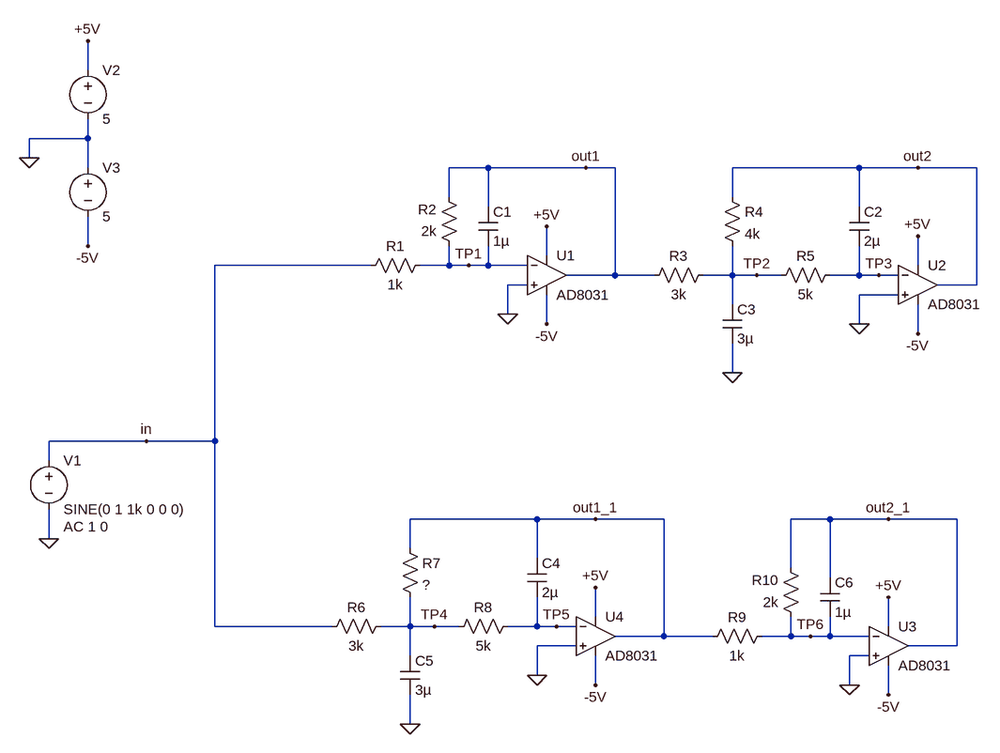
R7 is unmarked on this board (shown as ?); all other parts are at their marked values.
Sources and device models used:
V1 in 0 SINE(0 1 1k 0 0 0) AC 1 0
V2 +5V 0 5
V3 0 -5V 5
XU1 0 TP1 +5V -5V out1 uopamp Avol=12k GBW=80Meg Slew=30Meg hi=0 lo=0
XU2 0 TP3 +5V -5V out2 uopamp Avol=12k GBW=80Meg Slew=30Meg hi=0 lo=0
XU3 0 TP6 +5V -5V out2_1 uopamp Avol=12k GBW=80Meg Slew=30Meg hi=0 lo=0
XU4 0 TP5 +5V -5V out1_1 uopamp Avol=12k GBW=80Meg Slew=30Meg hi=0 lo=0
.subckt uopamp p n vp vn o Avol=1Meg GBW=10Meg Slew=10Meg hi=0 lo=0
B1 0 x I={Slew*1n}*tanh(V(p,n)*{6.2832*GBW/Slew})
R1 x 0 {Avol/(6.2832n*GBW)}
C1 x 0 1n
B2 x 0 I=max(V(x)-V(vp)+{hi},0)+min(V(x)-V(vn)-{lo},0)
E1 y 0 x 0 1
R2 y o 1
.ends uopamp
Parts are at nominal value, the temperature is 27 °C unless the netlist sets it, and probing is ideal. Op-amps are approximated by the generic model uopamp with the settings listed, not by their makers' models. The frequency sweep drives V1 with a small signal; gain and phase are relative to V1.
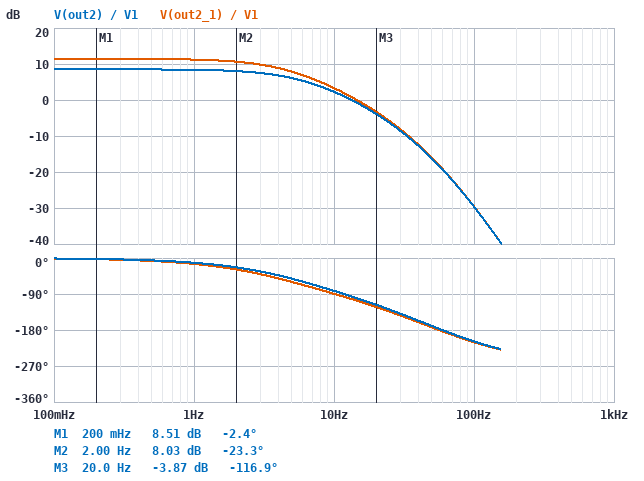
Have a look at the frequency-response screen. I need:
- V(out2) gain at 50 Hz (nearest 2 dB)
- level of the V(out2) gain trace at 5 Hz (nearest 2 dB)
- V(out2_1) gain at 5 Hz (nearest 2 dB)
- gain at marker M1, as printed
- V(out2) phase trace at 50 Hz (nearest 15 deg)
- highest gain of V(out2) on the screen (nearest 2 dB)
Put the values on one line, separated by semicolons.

-16 dB; 6 dB; 8 dB; 8.51 dB; -165 deg; 8 dB
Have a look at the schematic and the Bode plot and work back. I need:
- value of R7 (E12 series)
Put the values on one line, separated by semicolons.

5.6 kΩ
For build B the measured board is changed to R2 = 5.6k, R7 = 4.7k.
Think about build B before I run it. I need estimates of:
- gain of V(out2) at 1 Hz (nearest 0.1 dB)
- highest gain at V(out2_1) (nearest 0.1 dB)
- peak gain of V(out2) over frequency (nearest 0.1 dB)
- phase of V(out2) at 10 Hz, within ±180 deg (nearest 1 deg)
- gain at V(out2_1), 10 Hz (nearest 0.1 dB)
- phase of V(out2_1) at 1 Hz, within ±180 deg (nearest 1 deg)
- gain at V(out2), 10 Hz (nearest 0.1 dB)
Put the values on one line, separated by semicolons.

17.3 dB; 9.9 dB; 17.5 dB; -94 deg; 2.8 dB; -13 deg; 10.8 dB
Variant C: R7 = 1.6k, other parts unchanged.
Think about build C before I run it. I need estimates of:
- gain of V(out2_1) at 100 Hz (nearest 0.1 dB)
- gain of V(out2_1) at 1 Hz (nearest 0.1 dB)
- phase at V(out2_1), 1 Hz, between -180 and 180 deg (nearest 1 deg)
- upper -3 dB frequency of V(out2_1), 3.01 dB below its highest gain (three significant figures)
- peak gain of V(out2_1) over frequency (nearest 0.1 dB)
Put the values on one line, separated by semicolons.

-30.2 dB; 0.5 dB; -7 deg; 9.79 Hz; 0.6 dB
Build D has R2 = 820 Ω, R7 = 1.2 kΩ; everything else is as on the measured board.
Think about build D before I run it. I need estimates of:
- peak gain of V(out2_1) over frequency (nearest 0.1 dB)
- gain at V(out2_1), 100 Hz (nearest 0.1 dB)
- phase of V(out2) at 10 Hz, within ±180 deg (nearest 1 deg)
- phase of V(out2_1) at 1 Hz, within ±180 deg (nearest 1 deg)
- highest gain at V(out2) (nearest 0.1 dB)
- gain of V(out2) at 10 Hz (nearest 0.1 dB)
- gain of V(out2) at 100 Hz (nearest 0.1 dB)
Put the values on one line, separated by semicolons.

-1.9 dB; -30.5 dB; -78 deg; -7 deg; 0.8 dB; -5.4 dB; -34.3 dB
